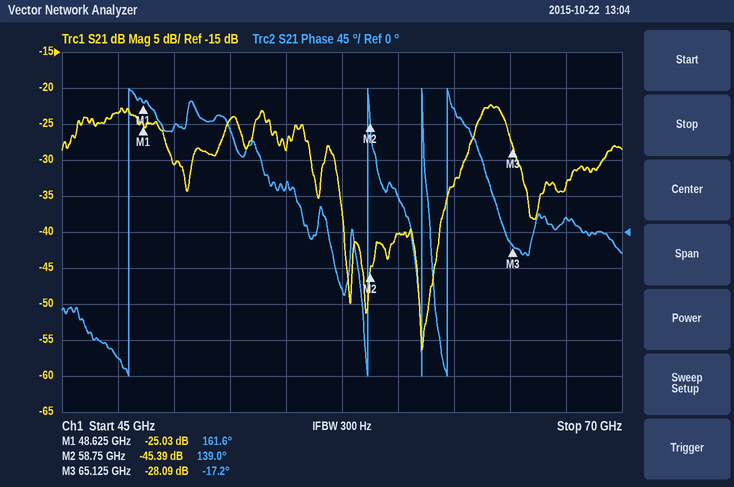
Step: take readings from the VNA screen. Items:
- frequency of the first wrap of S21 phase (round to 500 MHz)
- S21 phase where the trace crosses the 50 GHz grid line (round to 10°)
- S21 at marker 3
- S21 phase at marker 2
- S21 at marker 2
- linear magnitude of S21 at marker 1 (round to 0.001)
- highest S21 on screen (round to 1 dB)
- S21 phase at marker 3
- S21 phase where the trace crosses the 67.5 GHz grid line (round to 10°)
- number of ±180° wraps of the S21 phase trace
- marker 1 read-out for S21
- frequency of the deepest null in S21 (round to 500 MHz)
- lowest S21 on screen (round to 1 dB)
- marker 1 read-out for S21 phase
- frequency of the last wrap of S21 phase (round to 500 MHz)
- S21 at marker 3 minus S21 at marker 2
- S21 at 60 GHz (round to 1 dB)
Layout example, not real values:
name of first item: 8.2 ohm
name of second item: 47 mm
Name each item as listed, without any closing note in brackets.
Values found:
frequency of the first wrap of S21 phase: 48.0 GHz
S21 phase where the trace crosses the 50 GHz grid line: 130°
S21 at marker 3: -28.09 dB
S21 phase at marker 2: 139.0°
S21 at marker 2: -45.39 dB
linear magnitude of S21 at marker 1: 0.056
highest S21 on screen: -22 dB
S21 phase at marker 3: -17.2°
S21 phase where the trace crosses the 67.5 GHz grid line: 20°
number of ±180° wraps of the S21 phase trace: 4
marker 1 read-out for S21: -25.03 dB
frequency of the deepest null in S21: 61.0 GHz
lowest S21 on screen: -56 dB
marker 1 read-out for S21 phase: 161.6°
frequency of the last wrap of S21 phase: 62.0 GHz
S21 at marker 3 minus S21 at marker 2: 17.30 dB
S21 at 60 GHz: -40 dB
